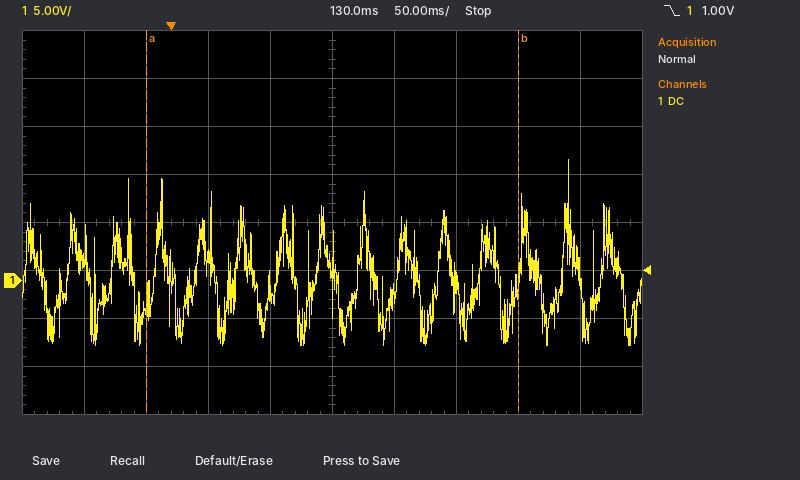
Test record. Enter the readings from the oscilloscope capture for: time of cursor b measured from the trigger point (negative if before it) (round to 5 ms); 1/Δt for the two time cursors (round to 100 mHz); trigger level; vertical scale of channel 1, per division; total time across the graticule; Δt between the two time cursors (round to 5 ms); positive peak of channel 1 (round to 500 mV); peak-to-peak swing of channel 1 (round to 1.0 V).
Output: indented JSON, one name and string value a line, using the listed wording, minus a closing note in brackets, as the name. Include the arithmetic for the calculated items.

{
  "time of cursor b measured from the trigger point (negative if before it)": "+280 ms",
  "1/Δt for the two time cursors": "1 / 300 ms ≈ 3.3 Hz",
  "trigger level": "1.00 V",
  "vertical scale of channel 1, per division": "5 V",
  "total time across the graticule": "500 ms",
  "Δt between the two time cursors": "300 ms",
  "positive peak of channel 1": "12.5 V",
  "peak-to-peak swing of channel 1": "19.0 V"
}
